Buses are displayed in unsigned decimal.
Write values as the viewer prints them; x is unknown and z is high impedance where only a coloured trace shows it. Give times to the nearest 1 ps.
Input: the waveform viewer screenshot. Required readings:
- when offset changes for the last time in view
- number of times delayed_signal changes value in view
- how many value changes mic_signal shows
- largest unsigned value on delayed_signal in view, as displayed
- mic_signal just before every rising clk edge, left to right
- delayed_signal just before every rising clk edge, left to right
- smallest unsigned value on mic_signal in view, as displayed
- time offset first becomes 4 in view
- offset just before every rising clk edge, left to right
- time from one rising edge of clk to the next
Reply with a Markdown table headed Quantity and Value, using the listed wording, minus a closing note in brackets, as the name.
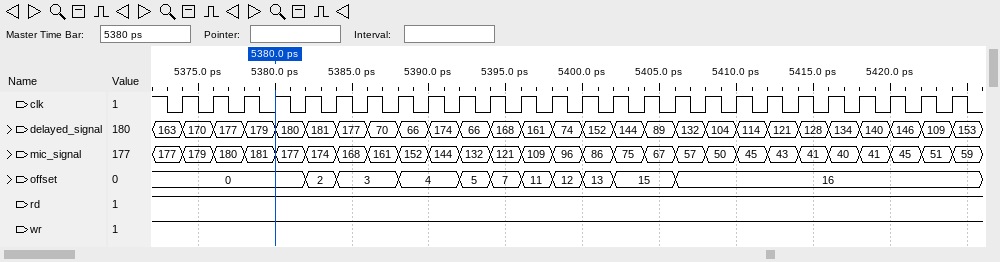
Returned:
| Quantity | Value |
|---|---|
| when offset changes for the last time in view | 5406 ps |
| number of times delayed_signal changes value in view | 26 |
| how many value changes mic_signal shows | 26 |
| largest unsigned value on delayed_signal in view, as displayed | 181 |
| mic_signal just before every rising clk edge, left to right | 177, 179, 180, 181, 177, 174, 168, 161, 152, 144, 132, 121, 109, 96, 86, 75, 67, 57, 50, 45, 43, 41, 40, 41, 45, 51 |
| delayed_signal just before every rising clk edge, left to right | 163, 170, 177, 179, 180, 181, 177, 70, 66, 174, 66, 168, 161, 74, 152, 144, 89, 132, 104, 114, 121, 128, 134, 140, 146, 109 |
| smallest unsigned value on mic_signal in view, as displayed | 40 |
| time offset first becomes 4 in view | 5388 ps |
| offset just before every rising clk edge, left to right | 0, 0, 0, 0, 0, 2, 3, 3, 4, 4, 5, 7, 11, 12, 13, 15, 15, 16, 16, 16, 16, 16, 16, 16, 16, 16 |
| time from one rising edge of clk to the next | 2 ps |
